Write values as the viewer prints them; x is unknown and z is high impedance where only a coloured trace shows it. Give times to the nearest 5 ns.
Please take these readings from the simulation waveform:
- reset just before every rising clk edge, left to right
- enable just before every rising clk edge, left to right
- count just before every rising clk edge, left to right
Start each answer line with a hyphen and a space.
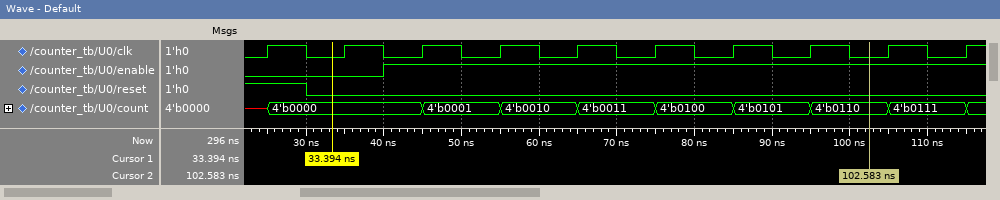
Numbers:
- 1 0 0 0 0 0 0 0 0 0
- 0 0 1 1 1 1 1 1 1 1
- x, 4'b0000, 4'b0000, 4'b0001, 4'b0010, 4'b0011, 4'b0100, 4'b0101, 4'b0110, 4'b0111
